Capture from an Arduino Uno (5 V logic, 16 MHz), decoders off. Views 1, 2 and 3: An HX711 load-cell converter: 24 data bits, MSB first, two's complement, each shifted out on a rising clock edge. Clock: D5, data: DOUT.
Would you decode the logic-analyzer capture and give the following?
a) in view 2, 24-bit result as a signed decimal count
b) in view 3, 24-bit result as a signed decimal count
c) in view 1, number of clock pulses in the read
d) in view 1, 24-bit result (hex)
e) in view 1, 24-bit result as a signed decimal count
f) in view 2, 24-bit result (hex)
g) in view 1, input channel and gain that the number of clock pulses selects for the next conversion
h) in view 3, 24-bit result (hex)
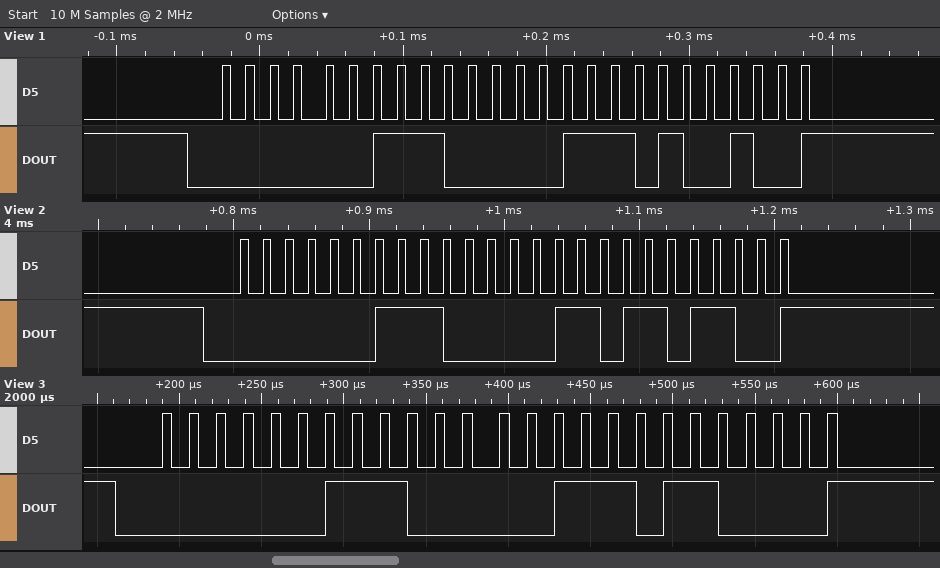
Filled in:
230252
230320
25
0x0383A4
230308
0x03836C
channel A, gain 128
0x0383B0
